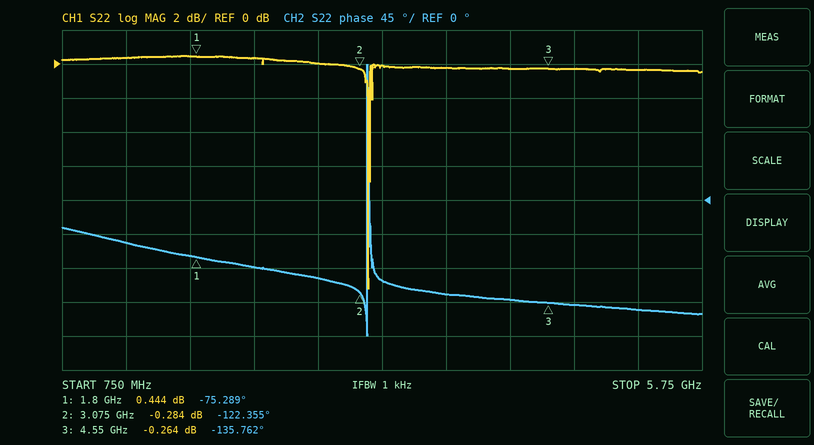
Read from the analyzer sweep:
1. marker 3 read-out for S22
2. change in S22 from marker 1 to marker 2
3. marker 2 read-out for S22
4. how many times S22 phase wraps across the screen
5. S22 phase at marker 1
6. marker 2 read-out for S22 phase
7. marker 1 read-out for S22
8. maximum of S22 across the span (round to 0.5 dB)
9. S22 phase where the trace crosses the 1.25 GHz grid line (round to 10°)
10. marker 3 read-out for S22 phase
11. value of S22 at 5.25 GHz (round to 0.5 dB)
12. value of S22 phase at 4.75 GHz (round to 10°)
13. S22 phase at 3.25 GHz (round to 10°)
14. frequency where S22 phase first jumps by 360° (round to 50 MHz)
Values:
-0.264 dB
-0.728 dB
-0.284 dB
1
-75.289°
-122.355°
0.444 dB
0.5 dB
-60°
-135.762°
-0.5 dB
-140°
-110°
3.15 GHz
